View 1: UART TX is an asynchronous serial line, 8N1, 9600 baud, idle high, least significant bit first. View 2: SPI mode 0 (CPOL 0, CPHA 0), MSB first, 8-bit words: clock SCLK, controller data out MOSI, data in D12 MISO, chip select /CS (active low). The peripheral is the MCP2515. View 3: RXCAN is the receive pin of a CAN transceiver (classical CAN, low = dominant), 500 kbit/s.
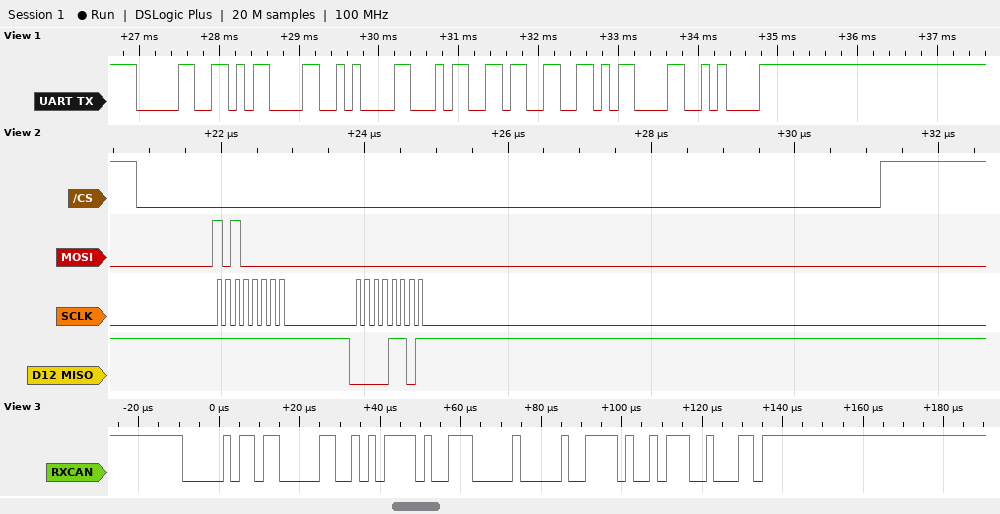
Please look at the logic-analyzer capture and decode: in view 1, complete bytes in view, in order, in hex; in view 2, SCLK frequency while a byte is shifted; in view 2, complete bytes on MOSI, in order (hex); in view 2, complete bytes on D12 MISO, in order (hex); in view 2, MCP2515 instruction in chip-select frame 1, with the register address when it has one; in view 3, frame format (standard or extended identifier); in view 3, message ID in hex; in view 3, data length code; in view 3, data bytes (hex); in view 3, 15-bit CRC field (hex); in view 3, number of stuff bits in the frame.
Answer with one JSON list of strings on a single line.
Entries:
["30 0D 0A 34 33 0D 0A", "8 MHz", "A0 00", "FF 0D", "READ STATUS", "standard", "0x036", "4", "AF 4E 00 1E", "0x4B91", "4"]
